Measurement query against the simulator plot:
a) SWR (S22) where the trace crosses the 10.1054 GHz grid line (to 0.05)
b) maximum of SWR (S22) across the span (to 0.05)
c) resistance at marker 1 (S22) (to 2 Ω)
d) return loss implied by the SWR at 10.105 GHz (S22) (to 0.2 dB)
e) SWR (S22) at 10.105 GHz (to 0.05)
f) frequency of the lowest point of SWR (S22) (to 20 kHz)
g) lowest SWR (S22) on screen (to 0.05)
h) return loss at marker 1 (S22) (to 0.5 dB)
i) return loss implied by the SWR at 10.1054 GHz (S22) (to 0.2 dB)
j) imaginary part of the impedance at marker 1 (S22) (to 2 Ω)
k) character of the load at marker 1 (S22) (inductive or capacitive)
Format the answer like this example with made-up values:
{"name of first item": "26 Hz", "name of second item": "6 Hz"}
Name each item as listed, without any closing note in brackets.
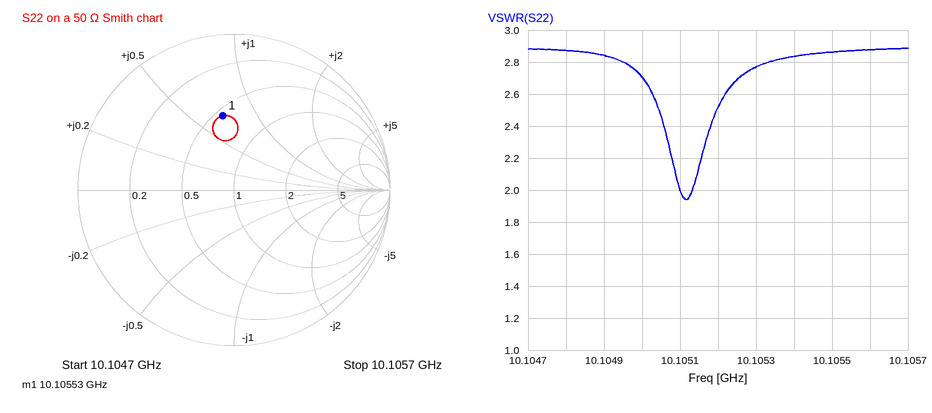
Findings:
{"SWR (S22) where the trace crosses the 10.1054 GHz grid line": "2.85", "maximum of SWR (S22) across the span": "2.90", "resistance at marker 1 (S22)": "28 Ω", "return loss implied by the SWR at 10.105 GHz (S22)": "6.8 dB", "SWR (S22) at 10.105 GHz": "2.70", "frequency of the lowest point of SWR (S22)": "10.10512 GHz", "lowest SWR (S22) on screen": "1.95", "return loss at marker 1 (S22)": "6.5 dB", "return loss implied by the SWR at 10.1054 GHz (S22)": "6.4 dB", "imaginary part of the impedance at marker 1 (S22)": "+34 Ω", "character of the load at marker 1 (S22)": "inductive"}
